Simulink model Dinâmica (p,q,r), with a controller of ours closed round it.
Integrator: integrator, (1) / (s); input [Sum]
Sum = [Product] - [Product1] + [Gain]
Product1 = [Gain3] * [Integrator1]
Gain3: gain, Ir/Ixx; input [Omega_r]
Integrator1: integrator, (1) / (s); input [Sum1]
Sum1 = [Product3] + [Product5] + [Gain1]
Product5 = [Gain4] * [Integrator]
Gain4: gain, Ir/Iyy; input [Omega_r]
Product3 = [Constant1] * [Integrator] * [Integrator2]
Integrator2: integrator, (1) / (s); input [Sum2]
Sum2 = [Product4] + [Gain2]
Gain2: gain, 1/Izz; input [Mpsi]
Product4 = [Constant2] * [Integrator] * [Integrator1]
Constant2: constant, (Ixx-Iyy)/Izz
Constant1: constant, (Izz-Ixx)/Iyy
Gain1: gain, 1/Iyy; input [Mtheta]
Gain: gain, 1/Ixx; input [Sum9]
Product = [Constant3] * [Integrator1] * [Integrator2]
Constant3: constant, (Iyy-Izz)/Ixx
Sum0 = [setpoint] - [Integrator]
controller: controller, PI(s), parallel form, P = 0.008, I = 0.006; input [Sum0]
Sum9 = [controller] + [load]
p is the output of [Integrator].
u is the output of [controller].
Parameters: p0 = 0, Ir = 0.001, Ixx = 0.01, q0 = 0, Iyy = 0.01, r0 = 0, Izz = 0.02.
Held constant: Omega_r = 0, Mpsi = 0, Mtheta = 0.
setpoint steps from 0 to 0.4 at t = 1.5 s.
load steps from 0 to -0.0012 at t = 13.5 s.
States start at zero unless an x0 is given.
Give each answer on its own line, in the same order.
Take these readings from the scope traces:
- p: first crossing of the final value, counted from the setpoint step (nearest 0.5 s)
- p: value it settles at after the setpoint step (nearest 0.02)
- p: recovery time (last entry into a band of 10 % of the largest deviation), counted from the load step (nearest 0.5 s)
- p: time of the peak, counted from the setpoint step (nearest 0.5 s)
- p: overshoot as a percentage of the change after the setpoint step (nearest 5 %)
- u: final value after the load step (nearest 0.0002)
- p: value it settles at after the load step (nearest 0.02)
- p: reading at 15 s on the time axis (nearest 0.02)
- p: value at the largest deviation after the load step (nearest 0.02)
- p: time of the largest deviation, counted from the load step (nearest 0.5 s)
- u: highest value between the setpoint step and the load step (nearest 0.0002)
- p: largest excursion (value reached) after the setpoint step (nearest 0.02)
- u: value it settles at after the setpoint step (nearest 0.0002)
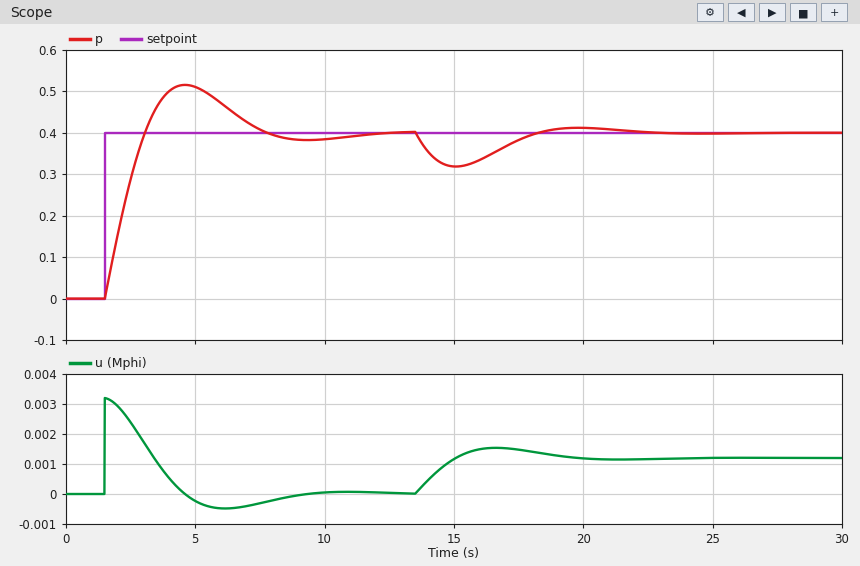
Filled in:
1.5 s
0.40
7.5 s
3.0 s
30 %
0.0012
0.40
0.32
0.32
1.5 s
0.0032
0.52
0.0000
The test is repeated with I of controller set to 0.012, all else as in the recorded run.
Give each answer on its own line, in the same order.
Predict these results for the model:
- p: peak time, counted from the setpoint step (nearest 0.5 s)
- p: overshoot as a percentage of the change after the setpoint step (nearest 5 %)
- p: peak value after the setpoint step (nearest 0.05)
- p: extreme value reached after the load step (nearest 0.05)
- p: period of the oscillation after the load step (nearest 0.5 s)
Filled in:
2.5 s
40 %
0.55
0.35
6.0 s
